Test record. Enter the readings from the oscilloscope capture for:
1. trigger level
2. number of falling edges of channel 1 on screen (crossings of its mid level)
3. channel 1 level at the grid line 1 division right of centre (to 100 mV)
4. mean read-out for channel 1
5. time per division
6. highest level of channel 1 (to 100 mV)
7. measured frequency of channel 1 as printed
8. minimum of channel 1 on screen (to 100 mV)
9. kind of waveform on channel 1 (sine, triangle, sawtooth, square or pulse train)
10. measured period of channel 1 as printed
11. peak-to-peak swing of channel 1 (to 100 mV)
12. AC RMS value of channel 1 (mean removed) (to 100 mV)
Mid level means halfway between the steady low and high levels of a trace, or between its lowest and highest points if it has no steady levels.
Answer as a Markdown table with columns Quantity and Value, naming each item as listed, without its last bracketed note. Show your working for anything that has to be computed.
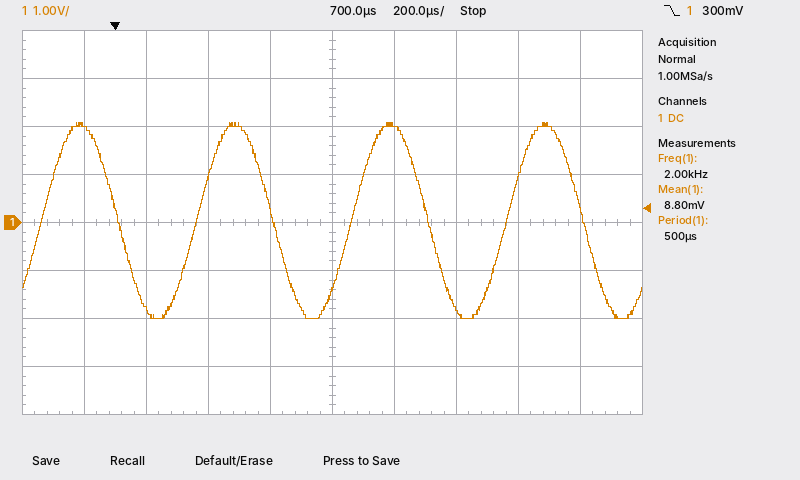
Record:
| Quantity | Value |
|---|---|
| trigger level | 300 mV |
| number of falling edges of channel 1 on screen | 4 |
| channel 1 level at the grid line 1 division right of centre | 2.0 V |
| mean read-out for channel 1 | 8.80 mV |
| time per division | 200 µs |
| highest level of channel 1 | 2.1 V |
| measured frequency of channel 1 as printed | 2.00 kHz |
| minimum of channel 1 on screen | -2.0 V |
| kind of waveform on channel 1 | sine |
| measured period of channel 1 as printed | 500 µs |
| peak-to-peak swing of channel 1 | 2.1 V − (-2.0 V) = 4.1 V |
| AC RMS value of channel 1 (mean removed) | 4.1 V / (2√2) ≈ 1.4 V |
